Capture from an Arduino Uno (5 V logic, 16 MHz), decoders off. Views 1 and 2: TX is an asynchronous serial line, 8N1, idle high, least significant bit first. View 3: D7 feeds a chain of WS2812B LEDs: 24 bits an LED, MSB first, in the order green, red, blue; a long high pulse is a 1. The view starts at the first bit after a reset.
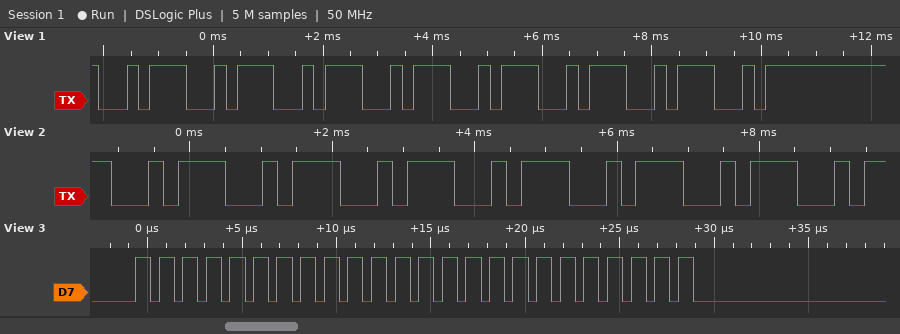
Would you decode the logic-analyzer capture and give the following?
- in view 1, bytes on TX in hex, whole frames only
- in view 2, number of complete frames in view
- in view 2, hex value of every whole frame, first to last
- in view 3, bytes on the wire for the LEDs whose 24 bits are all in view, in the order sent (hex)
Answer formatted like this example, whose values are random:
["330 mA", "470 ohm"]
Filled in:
["30 30 30 30 30 30 30 30", "7", "0x30 0x30 0x30 0x30 0x30 0x30 0x30", "FF FF FF"]
